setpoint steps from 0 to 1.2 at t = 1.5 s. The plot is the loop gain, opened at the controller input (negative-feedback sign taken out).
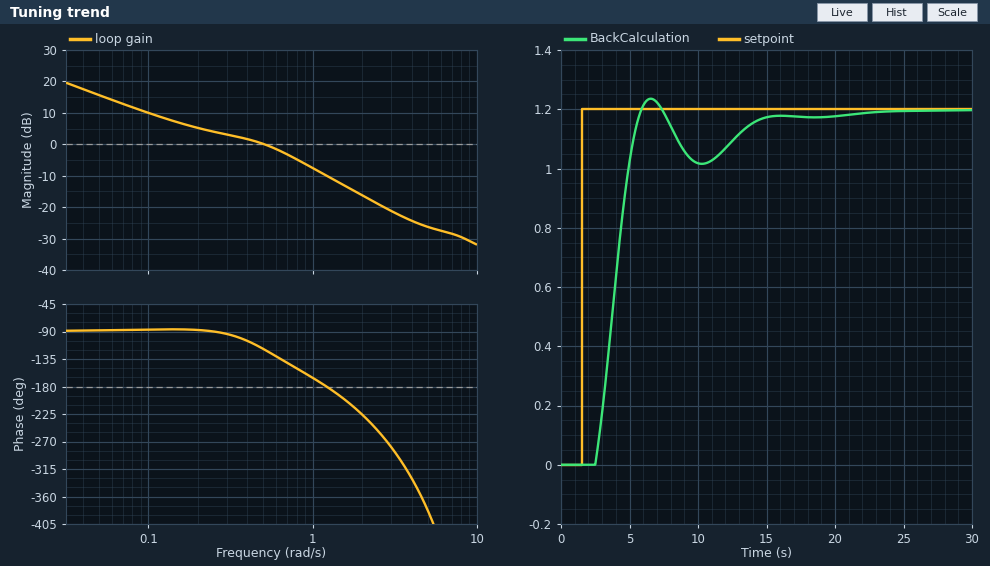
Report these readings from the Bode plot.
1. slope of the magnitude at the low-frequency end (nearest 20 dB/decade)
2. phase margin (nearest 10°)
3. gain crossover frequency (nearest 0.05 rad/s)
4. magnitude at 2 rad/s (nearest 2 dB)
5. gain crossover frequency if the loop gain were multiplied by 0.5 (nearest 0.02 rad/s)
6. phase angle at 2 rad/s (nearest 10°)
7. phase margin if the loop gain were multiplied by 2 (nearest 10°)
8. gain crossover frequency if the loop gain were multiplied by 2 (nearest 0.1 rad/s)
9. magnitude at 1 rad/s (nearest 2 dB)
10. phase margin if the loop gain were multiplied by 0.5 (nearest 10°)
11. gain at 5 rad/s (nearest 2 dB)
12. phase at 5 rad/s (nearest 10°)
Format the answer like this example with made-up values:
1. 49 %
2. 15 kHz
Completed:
1. -20 dB/decade
2. 60°
3. 0.50 rad/s
4. -16 dB
5. 0.18 rad/s
6. -230°
7. 20°
8. 0.9 rad/s
9. -8 dB
10. 90°
11. -26 dB
12. -380°
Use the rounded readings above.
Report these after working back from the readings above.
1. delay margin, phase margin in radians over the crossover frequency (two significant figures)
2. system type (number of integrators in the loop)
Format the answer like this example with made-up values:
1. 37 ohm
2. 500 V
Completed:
1. 2.1 s
2. 1
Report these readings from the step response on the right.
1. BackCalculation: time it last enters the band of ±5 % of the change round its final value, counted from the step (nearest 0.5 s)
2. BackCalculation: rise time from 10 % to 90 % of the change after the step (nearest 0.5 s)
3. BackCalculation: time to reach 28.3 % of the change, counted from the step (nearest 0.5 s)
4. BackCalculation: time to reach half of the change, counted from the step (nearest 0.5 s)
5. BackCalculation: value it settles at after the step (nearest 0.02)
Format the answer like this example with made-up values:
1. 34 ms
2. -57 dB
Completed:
1. 12.0 s
2. 2.5 s
3. 2.0 s
4. 2.5 s
5. 1.20
